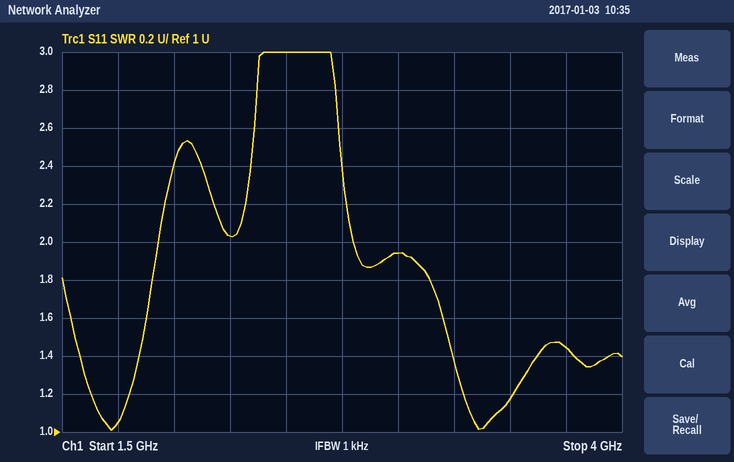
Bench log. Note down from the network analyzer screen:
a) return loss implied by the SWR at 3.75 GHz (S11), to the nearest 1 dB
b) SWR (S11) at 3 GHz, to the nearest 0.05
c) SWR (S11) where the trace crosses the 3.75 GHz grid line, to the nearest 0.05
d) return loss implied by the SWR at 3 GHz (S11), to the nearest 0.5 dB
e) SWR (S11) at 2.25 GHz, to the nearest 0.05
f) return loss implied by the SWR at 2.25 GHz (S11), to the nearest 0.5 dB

15 dB
1.95
1.45
10.0 dB
2.05
9.5 dB
